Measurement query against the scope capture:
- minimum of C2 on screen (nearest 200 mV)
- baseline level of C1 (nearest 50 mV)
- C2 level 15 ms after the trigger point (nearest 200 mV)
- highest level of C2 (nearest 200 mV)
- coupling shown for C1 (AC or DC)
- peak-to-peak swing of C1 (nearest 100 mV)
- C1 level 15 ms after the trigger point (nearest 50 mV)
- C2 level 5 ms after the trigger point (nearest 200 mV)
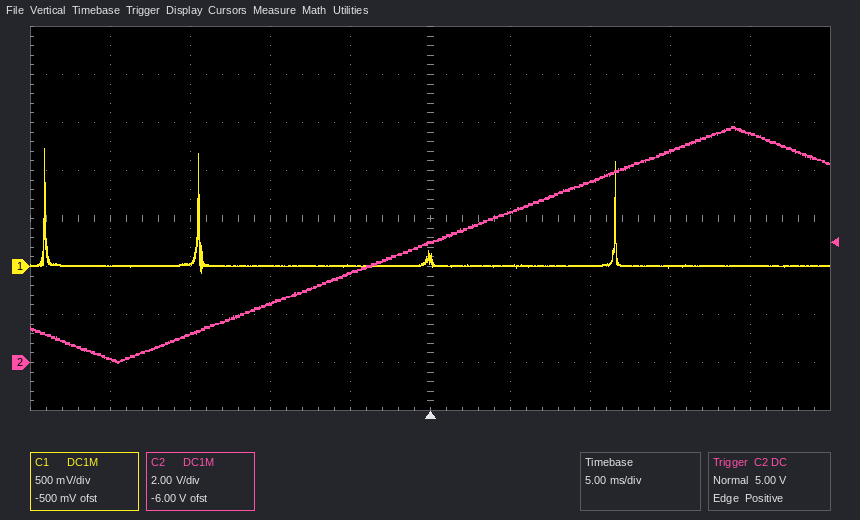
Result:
0.0 V
0 mV
8.8 V
9.8 V
DC
1.30 V
0 mV
6.2 V
